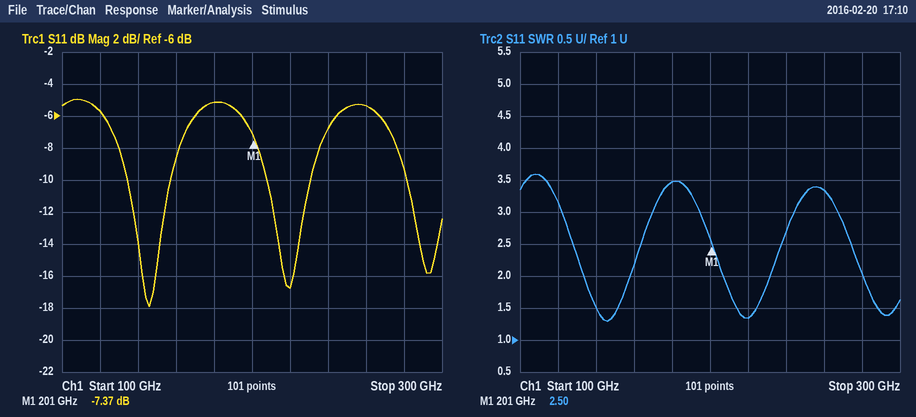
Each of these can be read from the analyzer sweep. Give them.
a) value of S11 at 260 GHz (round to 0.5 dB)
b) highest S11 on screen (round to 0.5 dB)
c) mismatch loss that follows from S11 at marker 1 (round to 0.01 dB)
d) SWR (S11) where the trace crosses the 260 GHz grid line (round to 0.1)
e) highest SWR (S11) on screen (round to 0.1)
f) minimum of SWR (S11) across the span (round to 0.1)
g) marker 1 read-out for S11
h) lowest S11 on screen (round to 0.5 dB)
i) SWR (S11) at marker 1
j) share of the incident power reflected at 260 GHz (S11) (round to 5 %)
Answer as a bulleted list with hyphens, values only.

- -5.5 dB
- -5.0 dB
- 0.88 dB
- 3.3
- 3.6
- 1.3
- -7.37 dB
- -18.0 dB
- 2.50
- 30 %
